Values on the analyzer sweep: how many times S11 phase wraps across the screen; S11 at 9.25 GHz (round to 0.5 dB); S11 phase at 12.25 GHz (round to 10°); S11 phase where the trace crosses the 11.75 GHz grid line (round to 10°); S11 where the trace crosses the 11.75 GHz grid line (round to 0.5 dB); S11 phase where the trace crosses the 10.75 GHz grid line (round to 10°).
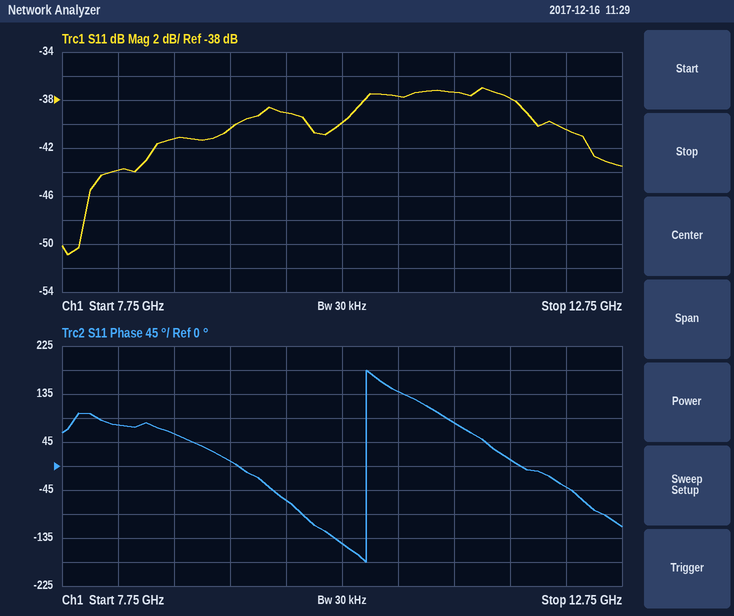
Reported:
1
-40.5 dB
-40°
10°
-38.0 dB
140°
